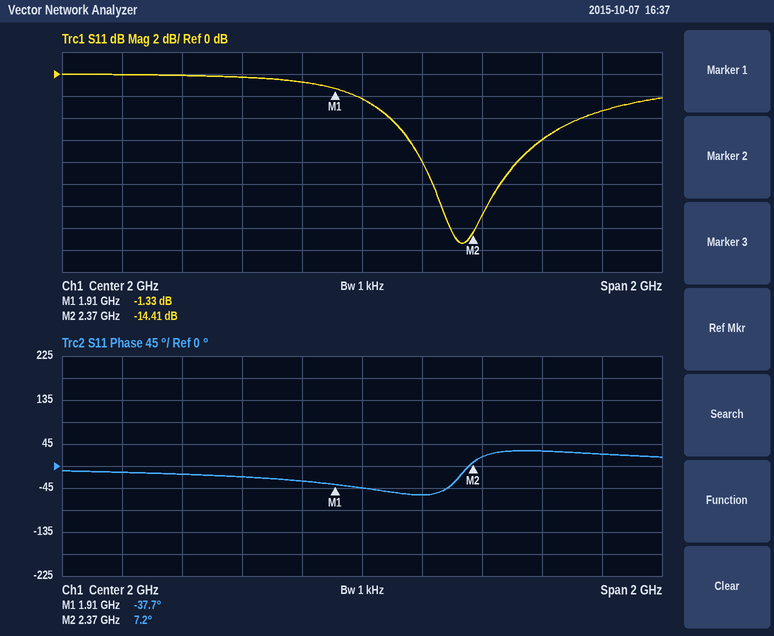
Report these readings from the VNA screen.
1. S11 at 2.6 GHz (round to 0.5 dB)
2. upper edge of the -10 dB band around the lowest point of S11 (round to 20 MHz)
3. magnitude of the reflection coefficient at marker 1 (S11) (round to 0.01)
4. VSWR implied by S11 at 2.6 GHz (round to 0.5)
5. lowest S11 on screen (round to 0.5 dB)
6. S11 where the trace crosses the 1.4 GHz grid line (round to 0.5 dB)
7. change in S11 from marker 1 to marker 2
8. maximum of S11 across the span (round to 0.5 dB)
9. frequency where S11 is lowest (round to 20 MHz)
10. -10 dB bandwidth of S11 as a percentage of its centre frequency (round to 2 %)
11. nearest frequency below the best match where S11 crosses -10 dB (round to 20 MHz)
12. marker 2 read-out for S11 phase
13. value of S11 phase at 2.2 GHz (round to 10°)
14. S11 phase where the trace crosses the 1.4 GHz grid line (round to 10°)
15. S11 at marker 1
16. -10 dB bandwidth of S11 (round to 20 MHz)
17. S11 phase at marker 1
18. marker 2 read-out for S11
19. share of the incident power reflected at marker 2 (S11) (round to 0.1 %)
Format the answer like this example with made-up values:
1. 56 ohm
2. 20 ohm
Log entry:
1. -6.0 dB
2. 2.46 GHz
3. 0.86
4. 3.0
5. -15.5 dB
6. 0.0 dB
7. -13.08 dB
8. 0.0 dB
9. 2.34 GHz
10. 10 %
11. 2.24 GHz
12. 7.2°
13. -60°
14. -20°
15. -1.33 dB
16. 220 MHz
17. -37.7°
18. -14.41 dB
19. 3.6 %
